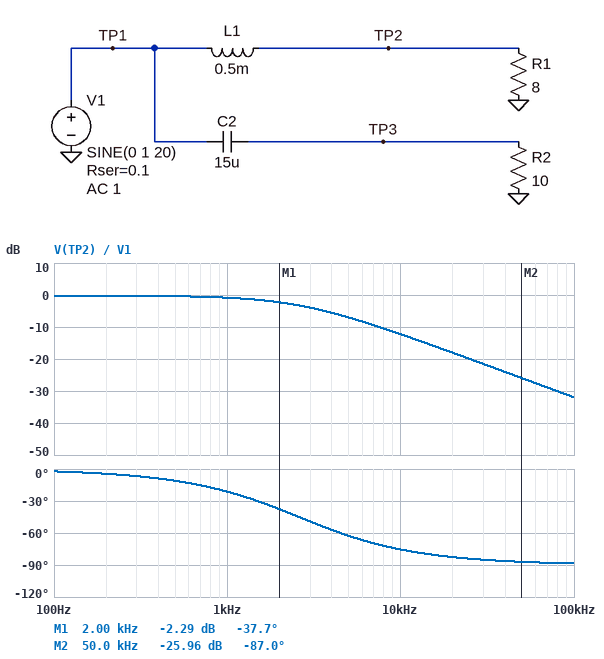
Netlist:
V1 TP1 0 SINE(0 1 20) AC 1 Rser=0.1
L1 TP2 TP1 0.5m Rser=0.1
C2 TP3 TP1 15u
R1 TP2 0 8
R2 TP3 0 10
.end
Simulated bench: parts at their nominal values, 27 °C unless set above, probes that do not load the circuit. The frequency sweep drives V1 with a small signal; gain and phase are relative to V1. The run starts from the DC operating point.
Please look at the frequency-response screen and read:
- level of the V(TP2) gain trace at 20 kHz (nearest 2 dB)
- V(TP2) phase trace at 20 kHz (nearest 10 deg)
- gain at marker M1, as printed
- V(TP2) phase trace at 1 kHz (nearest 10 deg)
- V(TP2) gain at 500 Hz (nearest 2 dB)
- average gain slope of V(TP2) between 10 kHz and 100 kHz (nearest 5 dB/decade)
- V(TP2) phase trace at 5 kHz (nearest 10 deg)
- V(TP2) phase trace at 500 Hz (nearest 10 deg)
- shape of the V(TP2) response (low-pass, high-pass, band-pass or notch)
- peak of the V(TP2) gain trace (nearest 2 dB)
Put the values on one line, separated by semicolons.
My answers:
-18 dB; -80 deg; -2.29 dB; -20 deg; 0 dB; -20 dB/decade; -60 deg; -10 deg; low-pass; 0 dB
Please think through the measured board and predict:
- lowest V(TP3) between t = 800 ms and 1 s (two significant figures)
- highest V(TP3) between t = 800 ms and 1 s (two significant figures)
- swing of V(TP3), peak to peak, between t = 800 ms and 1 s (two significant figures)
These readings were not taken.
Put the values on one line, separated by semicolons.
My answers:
-19 mV; 19 mV; 37 mV
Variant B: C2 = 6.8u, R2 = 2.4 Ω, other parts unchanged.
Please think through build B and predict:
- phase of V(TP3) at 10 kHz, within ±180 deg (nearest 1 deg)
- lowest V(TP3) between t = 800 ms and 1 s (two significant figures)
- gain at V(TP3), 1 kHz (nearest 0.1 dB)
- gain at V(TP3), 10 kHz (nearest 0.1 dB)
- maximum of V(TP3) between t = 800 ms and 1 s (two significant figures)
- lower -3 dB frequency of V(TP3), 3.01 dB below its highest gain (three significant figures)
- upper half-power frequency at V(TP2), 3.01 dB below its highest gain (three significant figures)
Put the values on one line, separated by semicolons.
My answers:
43 deg; -2.0 mV; -19.9 dB; -3.1 dB; 2.0 mV; 9.38 kHz; 2.60 kHz
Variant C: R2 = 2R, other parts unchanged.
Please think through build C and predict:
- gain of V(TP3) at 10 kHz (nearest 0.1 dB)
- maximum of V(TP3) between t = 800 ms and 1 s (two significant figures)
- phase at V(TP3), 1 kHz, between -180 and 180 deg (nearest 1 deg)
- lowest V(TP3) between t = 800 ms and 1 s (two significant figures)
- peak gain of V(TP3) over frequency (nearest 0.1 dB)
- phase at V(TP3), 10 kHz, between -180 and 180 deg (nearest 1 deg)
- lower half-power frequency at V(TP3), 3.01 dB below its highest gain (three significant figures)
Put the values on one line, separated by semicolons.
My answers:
-1.4 dB; 3.7 mV; 79 deg; -3.7 mV; -0.4 dB; 27 deg; 5.08 kHz
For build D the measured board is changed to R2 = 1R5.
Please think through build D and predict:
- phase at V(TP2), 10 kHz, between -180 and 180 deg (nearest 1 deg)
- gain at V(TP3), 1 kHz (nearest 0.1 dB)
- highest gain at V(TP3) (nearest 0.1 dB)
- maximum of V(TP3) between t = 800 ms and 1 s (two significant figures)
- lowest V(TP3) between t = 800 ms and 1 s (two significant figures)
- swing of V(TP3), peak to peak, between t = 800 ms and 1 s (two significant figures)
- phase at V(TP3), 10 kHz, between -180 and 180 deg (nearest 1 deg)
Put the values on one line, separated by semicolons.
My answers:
-77 deg; -17.2 dB; -0.6 dB; 2.8 mV; -2.8 mV; 5.6 mV; 34 deg
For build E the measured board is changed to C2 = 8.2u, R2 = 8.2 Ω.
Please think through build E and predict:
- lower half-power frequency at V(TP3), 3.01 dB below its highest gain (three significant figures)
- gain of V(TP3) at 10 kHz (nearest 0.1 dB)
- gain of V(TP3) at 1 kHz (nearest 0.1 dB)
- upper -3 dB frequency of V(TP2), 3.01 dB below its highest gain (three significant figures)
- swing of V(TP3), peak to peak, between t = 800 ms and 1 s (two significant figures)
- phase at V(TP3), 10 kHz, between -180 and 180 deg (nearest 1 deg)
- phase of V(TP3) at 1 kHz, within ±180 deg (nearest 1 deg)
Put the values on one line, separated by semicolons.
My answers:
2.37 kHz; -0.3 dB; -8.3 dB; 2.58 kHz; 17 mV; 13 deg; 67 deg
